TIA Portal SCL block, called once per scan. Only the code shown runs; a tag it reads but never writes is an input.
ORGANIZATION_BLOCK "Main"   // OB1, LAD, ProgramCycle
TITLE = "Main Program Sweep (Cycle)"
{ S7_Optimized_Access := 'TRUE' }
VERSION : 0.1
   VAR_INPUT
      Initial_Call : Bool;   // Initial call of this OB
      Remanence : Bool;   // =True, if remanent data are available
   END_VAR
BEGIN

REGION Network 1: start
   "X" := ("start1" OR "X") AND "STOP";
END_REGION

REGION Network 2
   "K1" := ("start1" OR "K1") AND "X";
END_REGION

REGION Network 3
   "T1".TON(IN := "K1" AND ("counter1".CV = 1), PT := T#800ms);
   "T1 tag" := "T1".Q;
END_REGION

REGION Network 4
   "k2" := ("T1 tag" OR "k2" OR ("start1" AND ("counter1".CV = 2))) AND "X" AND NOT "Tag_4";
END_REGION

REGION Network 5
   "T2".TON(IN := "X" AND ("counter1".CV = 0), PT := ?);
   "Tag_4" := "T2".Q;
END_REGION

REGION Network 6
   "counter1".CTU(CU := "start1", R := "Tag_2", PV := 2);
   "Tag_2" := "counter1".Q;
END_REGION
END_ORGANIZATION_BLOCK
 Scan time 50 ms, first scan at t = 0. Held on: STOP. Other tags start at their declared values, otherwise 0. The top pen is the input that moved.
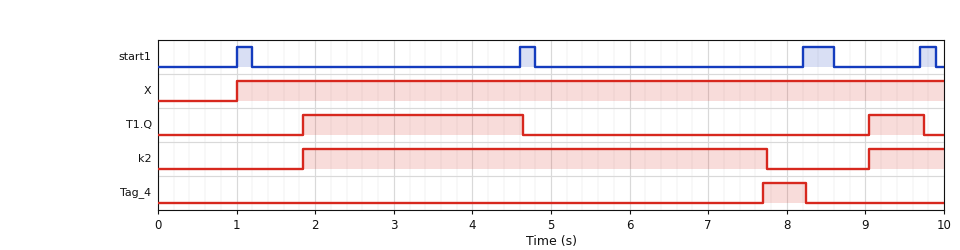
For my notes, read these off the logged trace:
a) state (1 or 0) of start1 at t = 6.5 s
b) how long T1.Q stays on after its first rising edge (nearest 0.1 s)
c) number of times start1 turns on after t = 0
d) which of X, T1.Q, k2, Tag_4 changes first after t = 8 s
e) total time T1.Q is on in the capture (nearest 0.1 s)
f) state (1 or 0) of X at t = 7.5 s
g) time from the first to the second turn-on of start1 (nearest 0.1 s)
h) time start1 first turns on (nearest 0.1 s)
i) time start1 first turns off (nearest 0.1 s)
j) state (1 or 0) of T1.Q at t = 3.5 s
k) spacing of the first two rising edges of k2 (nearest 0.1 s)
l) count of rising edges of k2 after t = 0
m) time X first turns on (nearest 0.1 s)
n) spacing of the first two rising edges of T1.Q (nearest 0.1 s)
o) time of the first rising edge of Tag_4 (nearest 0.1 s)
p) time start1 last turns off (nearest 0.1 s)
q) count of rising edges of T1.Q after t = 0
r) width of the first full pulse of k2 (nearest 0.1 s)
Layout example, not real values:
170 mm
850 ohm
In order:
0
2.8 s
4
Tag_4
3.5 s
1
3.6 s
1.0 s
1.2 s
1
7.2 s
2
1.0 s
7.2 s
7.7 s
9.9 s
2
5.9 s
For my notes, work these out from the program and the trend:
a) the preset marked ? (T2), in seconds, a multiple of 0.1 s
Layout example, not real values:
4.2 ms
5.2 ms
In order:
3.0 s
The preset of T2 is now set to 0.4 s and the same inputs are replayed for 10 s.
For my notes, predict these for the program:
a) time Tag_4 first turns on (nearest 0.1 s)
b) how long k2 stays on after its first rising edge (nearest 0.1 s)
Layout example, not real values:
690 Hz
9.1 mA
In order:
5.1 s
3.3 s
